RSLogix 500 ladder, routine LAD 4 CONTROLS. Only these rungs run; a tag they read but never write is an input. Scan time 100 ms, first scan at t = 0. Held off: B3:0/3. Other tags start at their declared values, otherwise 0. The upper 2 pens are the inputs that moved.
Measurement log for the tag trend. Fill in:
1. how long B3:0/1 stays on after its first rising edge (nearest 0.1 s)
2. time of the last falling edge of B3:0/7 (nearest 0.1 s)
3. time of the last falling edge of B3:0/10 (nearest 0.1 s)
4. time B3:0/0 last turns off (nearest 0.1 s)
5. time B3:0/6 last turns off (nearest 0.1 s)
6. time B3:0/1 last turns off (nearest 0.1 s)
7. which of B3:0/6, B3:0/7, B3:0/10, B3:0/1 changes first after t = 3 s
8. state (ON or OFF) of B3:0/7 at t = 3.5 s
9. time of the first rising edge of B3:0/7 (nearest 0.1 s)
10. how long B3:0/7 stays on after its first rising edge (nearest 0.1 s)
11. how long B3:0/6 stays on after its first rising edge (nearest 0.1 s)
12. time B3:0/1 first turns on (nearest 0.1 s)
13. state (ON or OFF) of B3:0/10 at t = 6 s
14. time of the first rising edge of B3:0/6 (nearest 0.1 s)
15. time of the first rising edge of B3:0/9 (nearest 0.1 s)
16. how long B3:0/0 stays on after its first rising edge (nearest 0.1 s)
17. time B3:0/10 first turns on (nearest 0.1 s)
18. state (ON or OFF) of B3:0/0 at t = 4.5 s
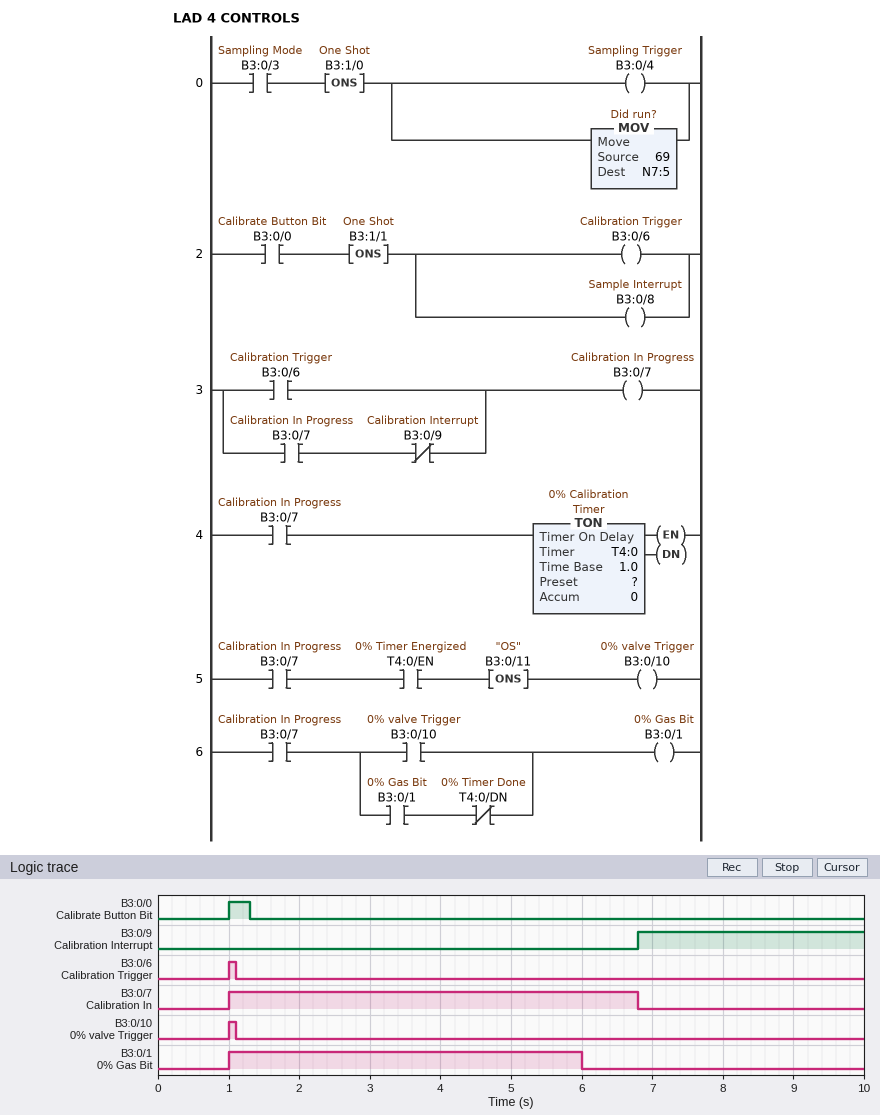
5.0 s
6.8 s
1.1 s
1.3 s
1.1 s
6.0 s
B3:0/1
ON
1.0 s
5.8 s
0.1 s
1.0 s
OFF
1.0 s
6.8 s
0.3 s
1.0 s
OFF
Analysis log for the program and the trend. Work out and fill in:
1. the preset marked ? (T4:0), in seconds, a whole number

5 s
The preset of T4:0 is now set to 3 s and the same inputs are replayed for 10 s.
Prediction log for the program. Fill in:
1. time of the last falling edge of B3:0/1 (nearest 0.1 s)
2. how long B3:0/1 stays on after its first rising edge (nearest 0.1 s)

4.0 s
3.0 s
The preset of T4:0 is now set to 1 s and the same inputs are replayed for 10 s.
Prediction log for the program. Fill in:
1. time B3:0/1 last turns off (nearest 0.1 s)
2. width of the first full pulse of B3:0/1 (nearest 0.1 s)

2.0 s
1.0 s
